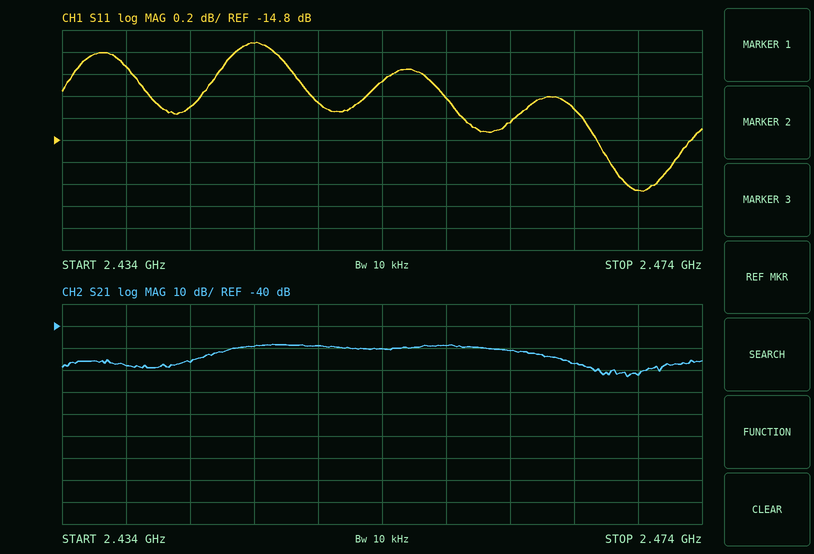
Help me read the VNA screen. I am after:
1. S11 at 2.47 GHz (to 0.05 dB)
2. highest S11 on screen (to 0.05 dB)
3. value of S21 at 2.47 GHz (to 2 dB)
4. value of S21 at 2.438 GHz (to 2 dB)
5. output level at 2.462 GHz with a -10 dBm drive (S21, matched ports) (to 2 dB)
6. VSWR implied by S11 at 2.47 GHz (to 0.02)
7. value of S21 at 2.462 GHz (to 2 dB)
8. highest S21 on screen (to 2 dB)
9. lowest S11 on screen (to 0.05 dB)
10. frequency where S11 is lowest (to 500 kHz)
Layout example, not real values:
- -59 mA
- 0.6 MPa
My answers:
- -15.25 dB
- -13.90 dB
- -62 dB
- -58 dB
- -62 dBm
- 1.42
- -52 dB
- -48 dB
- -15.25 dB
- 2.4705 GHz
